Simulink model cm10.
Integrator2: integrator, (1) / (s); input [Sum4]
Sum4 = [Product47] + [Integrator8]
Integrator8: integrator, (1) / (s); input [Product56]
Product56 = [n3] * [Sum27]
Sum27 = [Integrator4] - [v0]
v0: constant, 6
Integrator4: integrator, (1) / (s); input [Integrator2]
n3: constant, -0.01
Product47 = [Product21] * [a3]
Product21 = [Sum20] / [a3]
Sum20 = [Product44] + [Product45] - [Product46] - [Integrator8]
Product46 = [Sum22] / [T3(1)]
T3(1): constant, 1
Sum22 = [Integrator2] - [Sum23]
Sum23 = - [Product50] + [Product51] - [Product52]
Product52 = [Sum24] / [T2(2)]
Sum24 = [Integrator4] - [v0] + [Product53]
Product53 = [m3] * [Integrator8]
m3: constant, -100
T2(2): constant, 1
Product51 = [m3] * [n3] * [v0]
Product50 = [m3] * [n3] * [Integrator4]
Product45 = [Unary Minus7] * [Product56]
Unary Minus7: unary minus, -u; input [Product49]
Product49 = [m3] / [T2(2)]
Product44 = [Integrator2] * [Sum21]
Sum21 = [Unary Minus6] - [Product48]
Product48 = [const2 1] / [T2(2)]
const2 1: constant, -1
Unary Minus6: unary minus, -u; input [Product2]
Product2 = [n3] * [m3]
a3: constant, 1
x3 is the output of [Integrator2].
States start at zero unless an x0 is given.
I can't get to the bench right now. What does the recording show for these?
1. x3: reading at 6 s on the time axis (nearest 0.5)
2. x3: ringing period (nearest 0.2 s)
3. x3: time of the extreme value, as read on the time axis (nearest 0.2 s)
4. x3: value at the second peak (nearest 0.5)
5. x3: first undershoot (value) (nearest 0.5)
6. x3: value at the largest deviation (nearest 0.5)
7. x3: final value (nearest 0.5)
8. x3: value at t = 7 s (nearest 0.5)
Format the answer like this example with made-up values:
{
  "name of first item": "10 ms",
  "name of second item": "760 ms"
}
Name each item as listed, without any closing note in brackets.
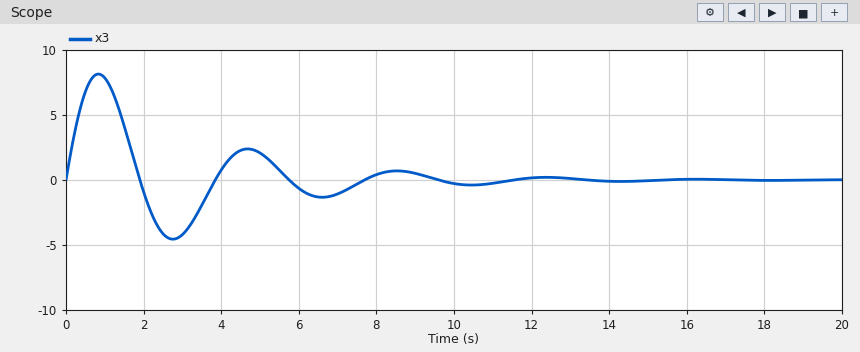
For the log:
{
  "x3: reading at 6 s on the time axis": "-0.5",
  "x3: ringing period": "3.8 s",
  "x3: time of the extreme value, as read on the time axis": "0.8 s",
  "x3: value at the second peak": "2.5",
  "x3: first undershoot (value)": "-4.5",
  "x3: value at the largest deviation": "8.0",
  "x3: final value": "0.0",
  "x3: value at t = 7 s": "-1.0"
}
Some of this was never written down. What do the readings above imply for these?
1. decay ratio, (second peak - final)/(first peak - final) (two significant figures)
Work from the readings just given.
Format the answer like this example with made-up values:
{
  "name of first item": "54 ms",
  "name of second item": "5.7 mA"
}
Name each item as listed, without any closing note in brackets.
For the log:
{
  "decay ratio, (second peak - final)/(first peak - final)": "0.31"
}
